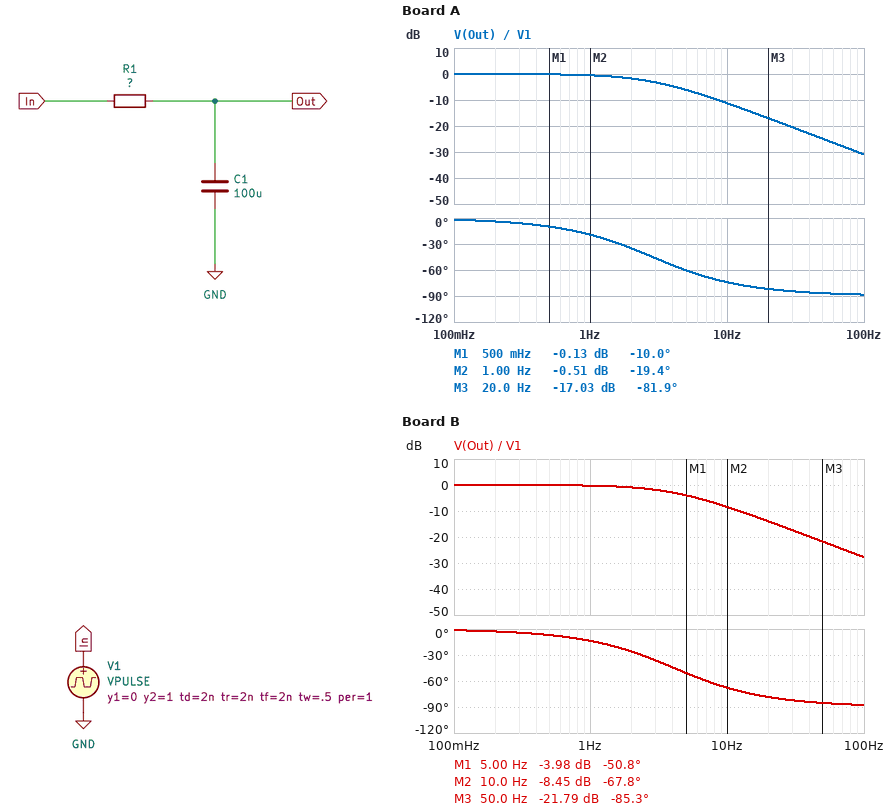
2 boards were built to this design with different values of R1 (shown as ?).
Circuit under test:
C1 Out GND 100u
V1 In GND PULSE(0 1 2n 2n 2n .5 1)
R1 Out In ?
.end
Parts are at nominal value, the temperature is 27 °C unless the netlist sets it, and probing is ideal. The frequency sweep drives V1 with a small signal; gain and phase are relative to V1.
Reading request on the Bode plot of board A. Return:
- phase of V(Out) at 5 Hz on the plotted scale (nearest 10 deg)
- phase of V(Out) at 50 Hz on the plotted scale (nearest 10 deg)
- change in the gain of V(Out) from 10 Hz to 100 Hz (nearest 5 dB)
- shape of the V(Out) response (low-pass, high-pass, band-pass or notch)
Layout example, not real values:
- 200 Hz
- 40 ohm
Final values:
- -60 deg
- -90 deg
- -20 dB
- low-pass
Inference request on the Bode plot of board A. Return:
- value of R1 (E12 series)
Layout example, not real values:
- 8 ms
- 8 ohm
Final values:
- 560 Ω
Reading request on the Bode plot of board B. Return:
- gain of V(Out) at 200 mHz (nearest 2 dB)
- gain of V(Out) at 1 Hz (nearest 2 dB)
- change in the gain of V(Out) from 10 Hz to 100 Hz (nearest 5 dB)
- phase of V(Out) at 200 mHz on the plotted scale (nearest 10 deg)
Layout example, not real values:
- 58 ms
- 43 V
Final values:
- 0 dB
- 0 dB
- -20 dB
- 0 deg
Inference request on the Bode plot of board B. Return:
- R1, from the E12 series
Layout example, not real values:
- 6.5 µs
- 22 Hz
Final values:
- 390 Ω
